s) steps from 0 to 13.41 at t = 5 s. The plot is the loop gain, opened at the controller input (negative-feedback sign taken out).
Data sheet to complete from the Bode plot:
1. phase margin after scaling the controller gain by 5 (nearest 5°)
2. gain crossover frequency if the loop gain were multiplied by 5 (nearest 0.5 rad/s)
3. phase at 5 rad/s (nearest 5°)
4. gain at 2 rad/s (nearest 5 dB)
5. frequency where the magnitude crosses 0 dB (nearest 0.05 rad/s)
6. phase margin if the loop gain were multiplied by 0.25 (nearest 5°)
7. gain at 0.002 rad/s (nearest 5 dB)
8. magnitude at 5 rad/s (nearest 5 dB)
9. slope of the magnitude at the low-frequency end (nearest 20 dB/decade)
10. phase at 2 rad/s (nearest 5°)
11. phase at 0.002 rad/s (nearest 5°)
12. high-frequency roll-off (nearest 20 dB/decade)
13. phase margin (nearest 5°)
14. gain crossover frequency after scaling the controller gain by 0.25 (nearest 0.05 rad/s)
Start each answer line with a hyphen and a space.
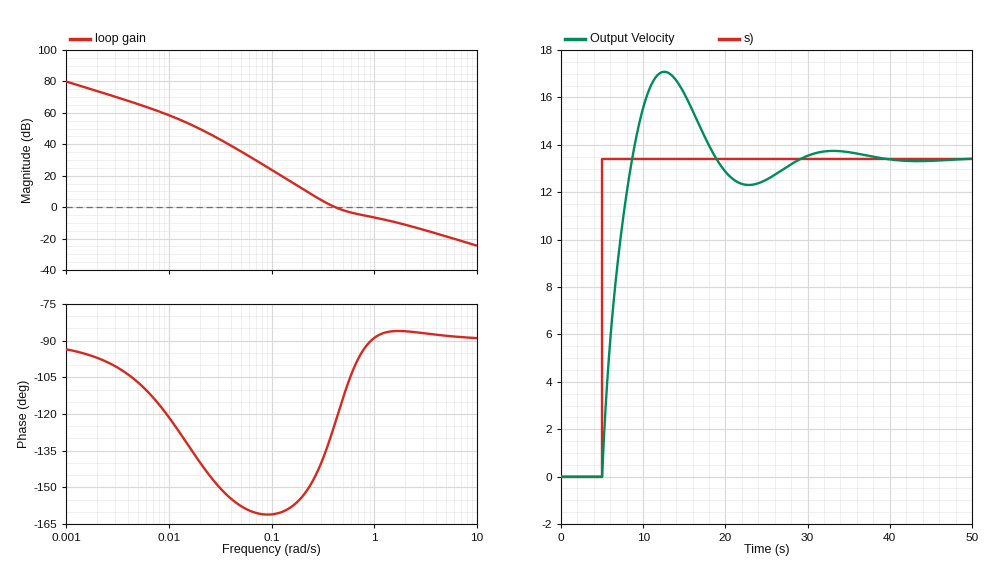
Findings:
- 95°
- 3.0 rad/s
- -90°
- -10 dB
- 0.40 rad/s
- 25°
- 75 dB
- -20 dB
- -20 dB/decade
- -85°
- -95°
- -20 dB/decade
- 55°
- 0.20 rad/s
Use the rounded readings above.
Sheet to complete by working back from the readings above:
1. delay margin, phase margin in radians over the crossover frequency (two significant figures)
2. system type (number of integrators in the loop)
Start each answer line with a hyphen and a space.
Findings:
- 2.4 s
- 1
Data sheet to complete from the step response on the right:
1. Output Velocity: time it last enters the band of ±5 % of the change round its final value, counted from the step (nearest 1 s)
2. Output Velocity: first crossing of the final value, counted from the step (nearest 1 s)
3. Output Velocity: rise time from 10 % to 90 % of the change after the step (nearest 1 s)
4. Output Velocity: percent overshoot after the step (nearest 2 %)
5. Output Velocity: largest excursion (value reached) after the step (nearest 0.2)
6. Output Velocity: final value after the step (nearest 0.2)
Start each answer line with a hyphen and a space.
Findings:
- 21 s
- 4 s
- 3 s
- 28 %
- 17.0
- 13.4
